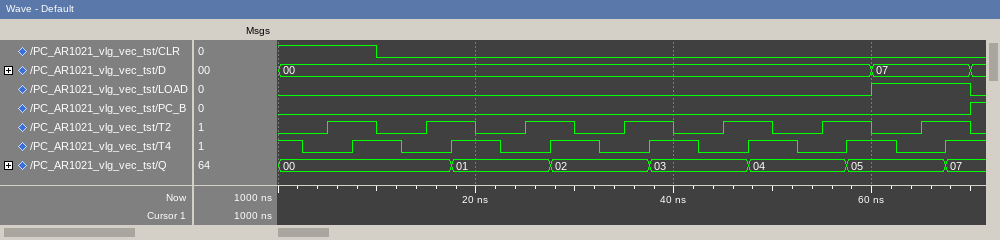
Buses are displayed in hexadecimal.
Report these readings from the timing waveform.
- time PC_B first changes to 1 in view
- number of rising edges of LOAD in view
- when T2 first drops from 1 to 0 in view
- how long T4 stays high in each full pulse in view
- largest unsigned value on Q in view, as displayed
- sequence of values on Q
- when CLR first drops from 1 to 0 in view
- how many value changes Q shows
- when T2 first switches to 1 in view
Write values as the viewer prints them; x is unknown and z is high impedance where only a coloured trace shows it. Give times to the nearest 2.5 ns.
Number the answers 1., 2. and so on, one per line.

1. 70 ns
2. 1
3. 10 ns
4. 5 ns, 5 ns, 5 ns, 5 ns, 5 ns, 5 ns
5. 07
6. 00, 01, 02, 03, 04, 05, 07
7. 10 ns
8. 6
9. 5 ns
